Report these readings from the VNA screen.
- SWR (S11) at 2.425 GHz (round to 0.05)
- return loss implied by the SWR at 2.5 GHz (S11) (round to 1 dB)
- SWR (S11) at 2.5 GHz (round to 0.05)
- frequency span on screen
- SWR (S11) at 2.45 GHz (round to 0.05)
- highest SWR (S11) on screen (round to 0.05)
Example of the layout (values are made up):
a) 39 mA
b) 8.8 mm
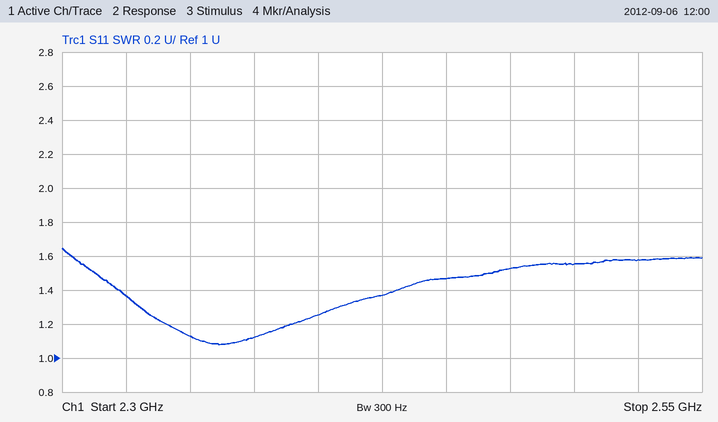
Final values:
a) 1.35
b) 13 dB
c) 1.55
d) 250 MHz
e) 1.45
f) 1.65
